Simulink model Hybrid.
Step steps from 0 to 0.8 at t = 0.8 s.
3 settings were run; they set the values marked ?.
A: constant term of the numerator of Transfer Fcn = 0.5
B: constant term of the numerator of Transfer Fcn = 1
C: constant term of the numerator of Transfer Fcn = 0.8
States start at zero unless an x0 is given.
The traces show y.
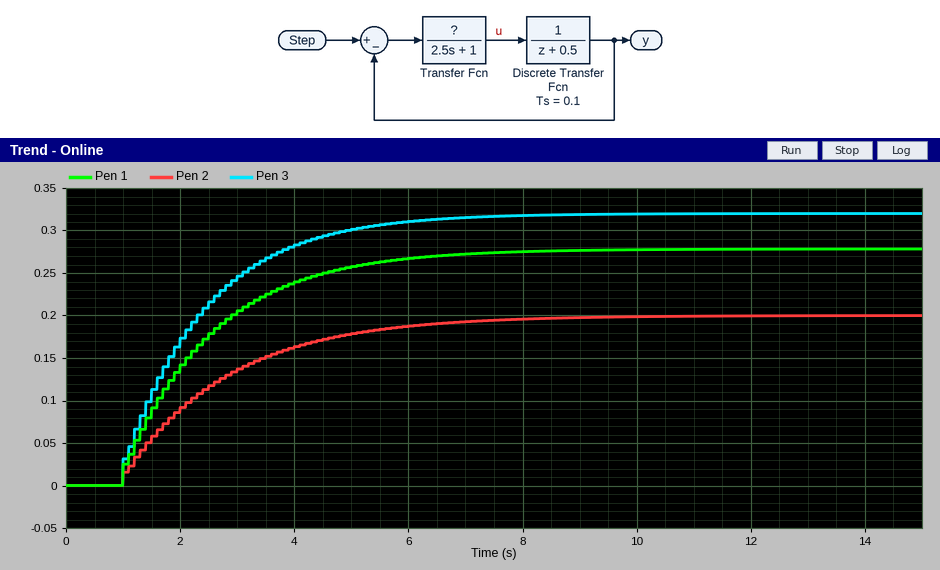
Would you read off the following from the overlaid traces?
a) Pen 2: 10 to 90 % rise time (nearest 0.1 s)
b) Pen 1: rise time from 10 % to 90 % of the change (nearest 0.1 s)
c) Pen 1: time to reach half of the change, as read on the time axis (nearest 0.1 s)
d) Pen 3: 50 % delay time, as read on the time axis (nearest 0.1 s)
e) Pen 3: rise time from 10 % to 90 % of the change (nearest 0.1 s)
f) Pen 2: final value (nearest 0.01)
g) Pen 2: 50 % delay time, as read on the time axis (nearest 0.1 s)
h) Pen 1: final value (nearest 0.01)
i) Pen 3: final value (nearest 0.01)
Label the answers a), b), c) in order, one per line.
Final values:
a) 4.1 s
b) 3.5 s
c) 2.0 s
d) 1.9 s
e) 3.2 s
f) 0.20
g) 2.2 s
h) 0.28
i) 0.32
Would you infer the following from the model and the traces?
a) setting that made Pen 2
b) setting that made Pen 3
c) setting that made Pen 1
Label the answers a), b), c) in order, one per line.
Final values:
a) A
b) B
c) C
